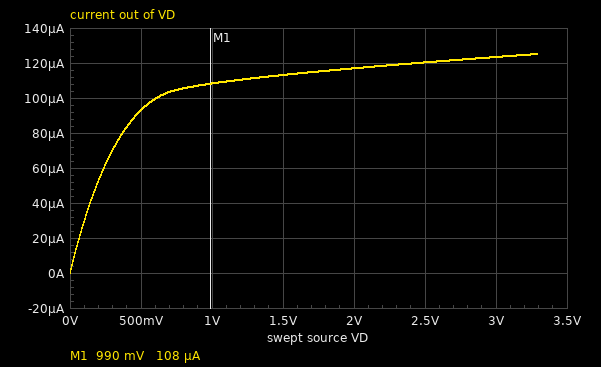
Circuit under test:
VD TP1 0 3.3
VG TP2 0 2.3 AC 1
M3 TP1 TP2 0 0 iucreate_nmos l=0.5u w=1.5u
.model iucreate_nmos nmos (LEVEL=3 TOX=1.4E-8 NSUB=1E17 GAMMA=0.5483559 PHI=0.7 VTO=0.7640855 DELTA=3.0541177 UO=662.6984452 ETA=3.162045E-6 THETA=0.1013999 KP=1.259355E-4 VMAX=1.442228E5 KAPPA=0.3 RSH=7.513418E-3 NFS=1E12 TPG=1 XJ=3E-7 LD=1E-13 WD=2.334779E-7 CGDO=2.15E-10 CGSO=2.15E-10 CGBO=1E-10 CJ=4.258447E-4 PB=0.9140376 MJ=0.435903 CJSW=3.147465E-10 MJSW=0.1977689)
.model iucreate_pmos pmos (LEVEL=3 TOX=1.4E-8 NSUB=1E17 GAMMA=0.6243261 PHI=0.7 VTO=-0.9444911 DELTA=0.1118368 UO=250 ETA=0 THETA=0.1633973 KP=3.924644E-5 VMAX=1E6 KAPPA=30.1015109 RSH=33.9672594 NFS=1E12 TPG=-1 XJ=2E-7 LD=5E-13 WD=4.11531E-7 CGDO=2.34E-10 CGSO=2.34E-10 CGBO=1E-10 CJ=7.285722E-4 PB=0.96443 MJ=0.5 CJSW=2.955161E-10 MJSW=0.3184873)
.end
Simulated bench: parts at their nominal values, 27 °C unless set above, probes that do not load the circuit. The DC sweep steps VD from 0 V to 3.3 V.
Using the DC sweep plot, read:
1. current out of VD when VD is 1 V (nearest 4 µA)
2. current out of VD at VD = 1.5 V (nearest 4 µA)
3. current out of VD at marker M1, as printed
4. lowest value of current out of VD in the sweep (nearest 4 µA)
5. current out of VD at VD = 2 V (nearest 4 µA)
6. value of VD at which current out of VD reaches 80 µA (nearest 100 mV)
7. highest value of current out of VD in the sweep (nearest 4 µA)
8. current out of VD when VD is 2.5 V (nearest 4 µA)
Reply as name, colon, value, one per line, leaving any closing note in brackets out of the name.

current out of VD when VD is 1 V: 108 µA
current out of VD at VD = 1.5 V: 112 µA
current out of VD at marker M1, as printed: 108 µA
lowest value of current out of VD in the sweep: 0 A
current out of VD at VD = 2 V: 116 µA
value of VD at which current out of VD reaches 80 µA: 400 mV
highest value of current out of VD in the sweep: 124 µA
current out of VD when VD is 2.5 V: 120 µA
